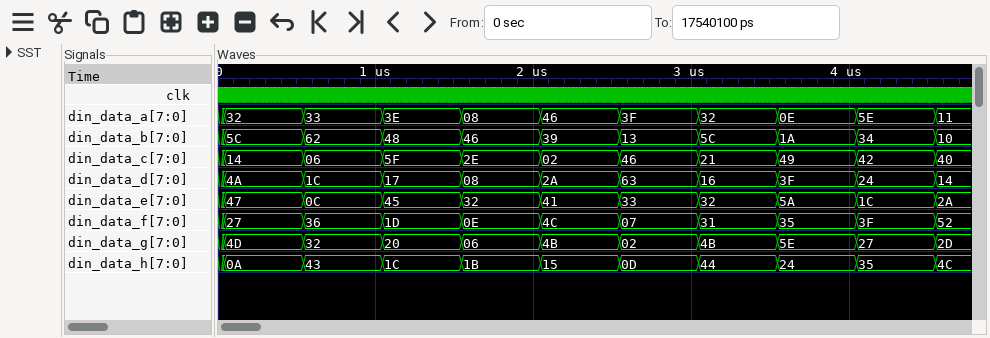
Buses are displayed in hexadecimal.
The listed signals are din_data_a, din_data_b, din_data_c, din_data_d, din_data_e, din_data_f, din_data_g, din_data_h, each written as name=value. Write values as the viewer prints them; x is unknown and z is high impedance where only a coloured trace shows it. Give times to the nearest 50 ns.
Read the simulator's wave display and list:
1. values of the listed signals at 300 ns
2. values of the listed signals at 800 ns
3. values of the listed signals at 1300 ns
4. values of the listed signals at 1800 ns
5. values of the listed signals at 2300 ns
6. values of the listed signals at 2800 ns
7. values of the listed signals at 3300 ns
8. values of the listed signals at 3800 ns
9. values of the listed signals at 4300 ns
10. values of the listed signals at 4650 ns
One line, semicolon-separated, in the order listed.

din_data_a=32, din_data_b=5C, din_data_c=14, din_data_d=4A, din_data_e=47, din_data_f=27, din_data_g=4D, din_data_h=0A; din_data_a=33, din_data_b=62, din_data_c=06, din_data_d=1C, din_data_e=0C, din_data_f=36, din_data_g=32, din_data_h=43; din_data_a=3E, din_data_b=48, din_data_c=5F, din_data_d=17, din_data_e=45, din_data_f=1D, din_data_g=20, din_data_h=1C; din_data_a=08, din_data_b=46, din_data_c=2E, din_data_d=08, din_data_e=32, din_data_f=0E, din_data_g=06, din_data_h=1B; din_data_a=46, din_data_b=39, din_data_c=02, din_data_d=2A, din_data_e=41, din_data_f=4C, din_data_g=4B, din_data_h=15; din_data_a=3F, din_data_b=13, din_data_c=46, din_data_d=63, din_data_e=33, din_data_f=07, din_data_g=02, din_data_h=0D; din_data_a=32, din_data_b=5C, din_data_c=21, din_data_d=16, din_data_e=32, din_data_f=31, din_data_g=4B, din_data_h=44; din_data_a=0E, din_data_b=1A, din_data_c=49, din_data_d=3F, din_data_e=5A, din_data_f=35, din_data_g=5E, din_data_h=24; din_data_a=5E, din_data_b=34, din_data_c=42, din_data_d=24, din_data_e=1C, din_data_f=3F, din_data_g=27, din_data_h=35; din_data_a=11, din_data_b=10, din_data_c=40, din_data_d=14, din_data_e=2A, din_data_f=52, din_data_g=2D, din_data_h=4C
